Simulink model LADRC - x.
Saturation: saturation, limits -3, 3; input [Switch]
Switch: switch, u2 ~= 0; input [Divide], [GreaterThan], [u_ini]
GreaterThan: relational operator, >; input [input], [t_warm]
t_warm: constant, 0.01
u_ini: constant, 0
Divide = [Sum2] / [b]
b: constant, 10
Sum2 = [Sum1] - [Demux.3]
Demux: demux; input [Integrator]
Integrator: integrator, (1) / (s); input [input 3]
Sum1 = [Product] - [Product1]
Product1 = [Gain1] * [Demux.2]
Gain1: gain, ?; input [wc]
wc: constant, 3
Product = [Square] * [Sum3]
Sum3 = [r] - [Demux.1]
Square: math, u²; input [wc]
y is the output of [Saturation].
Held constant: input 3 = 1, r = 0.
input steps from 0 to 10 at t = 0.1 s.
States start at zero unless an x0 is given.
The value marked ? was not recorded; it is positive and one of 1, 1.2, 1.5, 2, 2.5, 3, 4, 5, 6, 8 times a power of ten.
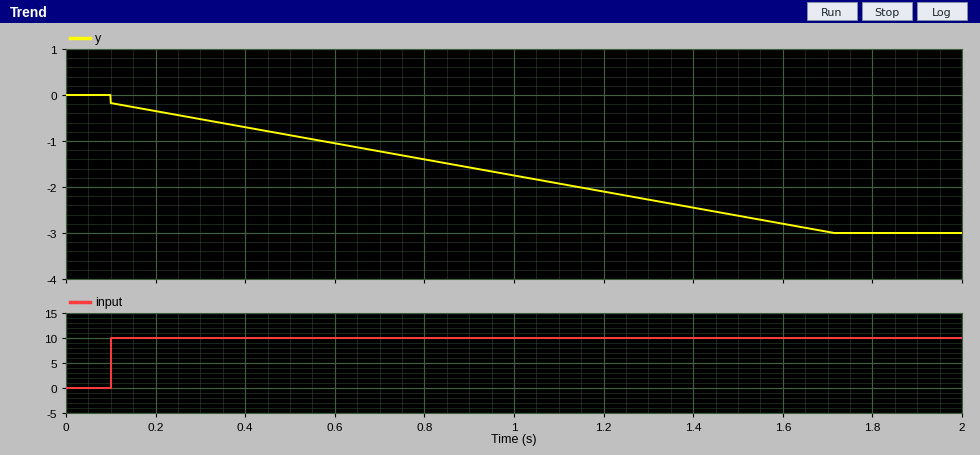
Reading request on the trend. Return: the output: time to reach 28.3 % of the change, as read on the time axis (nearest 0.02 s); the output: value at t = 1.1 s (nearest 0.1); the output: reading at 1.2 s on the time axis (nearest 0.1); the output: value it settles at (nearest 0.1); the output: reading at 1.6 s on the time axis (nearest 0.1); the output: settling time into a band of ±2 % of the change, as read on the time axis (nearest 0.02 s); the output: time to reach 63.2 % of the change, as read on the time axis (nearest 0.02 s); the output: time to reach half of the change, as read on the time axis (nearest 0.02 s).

0.48 s
-1.9
-2.1
-3.0
-2.8
1.68 s
1.08 s
0.86 s
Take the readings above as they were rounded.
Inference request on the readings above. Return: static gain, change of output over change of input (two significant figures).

-0.30
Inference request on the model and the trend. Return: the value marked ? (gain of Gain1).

2.5
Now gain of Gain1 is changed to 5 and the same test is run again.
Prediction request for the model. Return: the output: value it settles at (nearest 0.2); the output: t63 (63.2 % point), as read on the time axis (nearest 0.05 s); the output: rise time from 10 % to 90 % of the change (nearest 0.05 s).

-3.0
0.75 s
0.95 s
